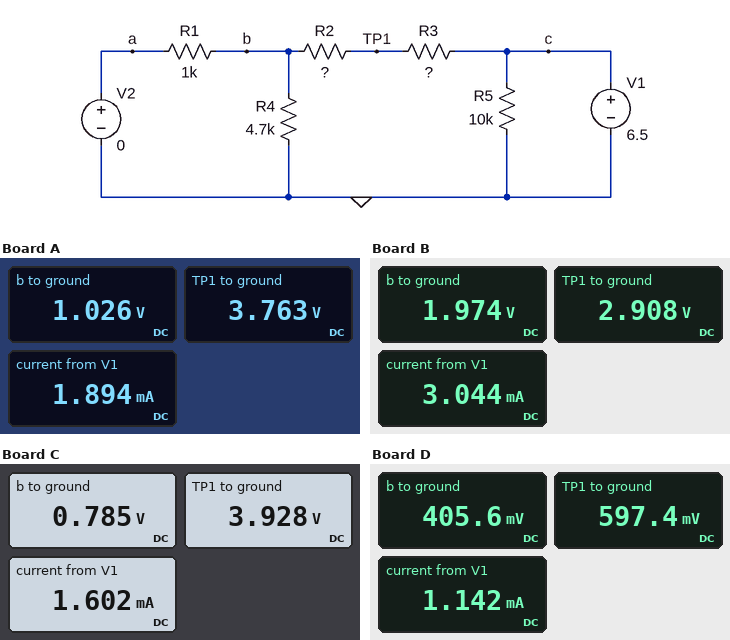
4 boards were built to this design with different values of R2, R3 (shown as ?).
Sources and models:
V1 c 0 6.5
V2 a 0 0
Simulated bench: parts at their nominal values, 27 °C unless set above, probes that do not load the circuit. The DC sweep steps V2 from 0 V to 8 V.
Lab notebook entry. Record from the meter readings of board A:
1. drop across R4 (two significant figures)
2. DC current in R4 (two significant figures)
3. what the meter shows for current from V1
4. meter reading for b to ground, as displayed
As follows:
1.0 V
220 µA
1.894 mA
1.026 V
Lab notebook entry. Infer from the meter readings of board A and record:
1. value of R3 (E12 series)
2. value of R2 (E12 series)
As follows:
2.2 kΩ
2.2 kΩ
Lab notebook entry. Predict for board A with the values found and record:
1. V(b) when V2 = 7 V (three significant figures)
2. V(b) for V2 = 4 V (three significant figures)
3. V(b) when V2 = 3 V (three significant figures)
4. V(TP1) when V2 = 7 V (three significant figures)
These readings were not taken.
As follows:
5.89 V
3.80 V
3.11 V
6.19 V
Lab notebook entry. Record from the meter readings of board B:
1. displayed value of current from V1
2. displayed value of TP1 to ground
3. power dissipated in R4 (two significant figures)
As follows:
3.044 mA
2.908 V
830 µW
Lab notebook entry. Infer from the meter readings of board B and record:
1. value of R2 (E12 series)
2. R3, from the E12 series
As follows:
390 Ω
1.5 kΩ
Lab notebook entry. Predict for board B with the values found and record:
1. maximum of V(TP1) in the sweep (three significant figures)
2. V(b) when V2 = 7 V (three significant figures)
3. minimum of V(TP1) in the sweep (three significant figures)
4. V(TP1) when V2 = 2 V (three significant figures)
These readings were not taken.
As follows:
6.55 V
5.99 V
2.91 V
3.82 V
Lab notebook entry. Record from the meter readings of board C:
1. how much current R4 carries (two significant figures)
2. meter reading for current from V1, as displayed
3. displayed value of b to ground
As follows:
170 µA
1.602 mA
0.785 V
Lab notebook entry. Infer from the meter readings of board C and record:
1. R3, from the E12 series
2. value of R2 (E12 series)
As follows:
2.7 kΩ
3.3 kΩ
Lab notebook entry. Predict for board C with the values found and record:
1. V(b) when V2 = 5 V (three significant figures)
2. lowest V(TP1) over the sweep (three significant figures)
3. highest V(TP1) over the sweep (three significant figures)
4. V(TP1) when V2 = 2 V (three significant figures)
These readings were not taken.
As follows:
4.41 V
3.93 V
6.54 V
4.58 V
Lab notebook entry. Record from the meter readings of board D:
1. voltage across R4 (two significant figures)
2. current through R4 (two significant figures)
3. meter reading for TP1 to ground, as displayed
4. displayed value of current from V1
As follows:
410 mV
86 µA
597.4 mV
1.142 mA
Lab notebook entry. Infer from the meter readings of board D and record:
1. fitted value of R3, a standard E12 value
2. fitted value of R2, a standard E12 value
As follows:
12 kΩ
390 Ω
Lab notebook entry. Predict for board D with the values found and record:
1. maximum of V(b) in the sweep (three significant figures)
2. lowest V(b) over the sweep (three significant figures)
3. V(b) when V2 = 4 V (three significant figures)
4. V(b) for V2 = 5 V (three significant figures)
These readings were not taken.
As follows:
6.59 V
406 mV
3.50 V
4.27 V
